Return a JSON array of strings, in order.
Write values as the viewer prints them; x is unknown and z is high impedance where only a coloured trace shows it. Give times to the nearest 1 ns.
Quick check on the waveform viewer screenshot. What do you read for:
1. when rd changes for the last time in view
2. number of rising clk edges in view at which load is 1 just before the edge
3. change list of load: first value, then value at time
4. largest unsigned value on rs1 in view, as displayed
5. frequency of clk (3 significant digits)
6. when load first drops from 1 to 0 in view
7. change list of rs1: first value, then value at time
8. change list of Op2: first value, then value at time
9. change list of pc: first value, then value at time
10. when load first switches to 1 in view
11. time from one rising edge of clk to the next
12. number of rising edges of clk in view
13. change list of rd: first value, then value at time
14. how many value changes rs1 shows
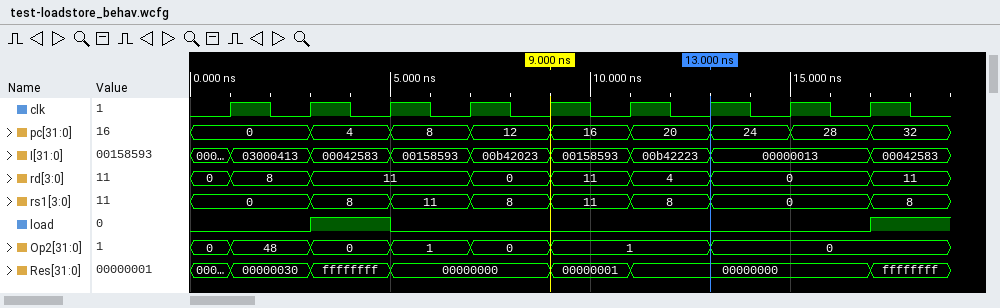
["17 ns", "1", "0, 1 at 3 ns, 0 at 5 ns, 1 at 17 ns", "11", "500 MHz", "5 ns", "0, 8 at 3 ns, 11 at 5 ns, 8 at 7 ns, 11 at 9 ns, 8 at 11 ns, 0 at 13 ns, 8 at 17 ns", "0, 48 at 1 ns, 0 at 3 ns, 1 at 5 ns, 0 at 7 ns, 1 at 9 ns, 0 at 13 ns", "0, 4 at 3 ns, 8 at 5 ns, 12 at 7 ns, 16 at 9 ns, 20 at 11 ns, 24 at 13 ns, 28 at 15 ns, 32 at 17 ns", "3 ns", "2 ns", "9", "0, 8 at 1 ns, 11 at 3 ns, 0 at 7 ns, 11 at 9 ns, 4 at 11 ns, 0 at 13 ns, 11 at 17 ns", "7"]
